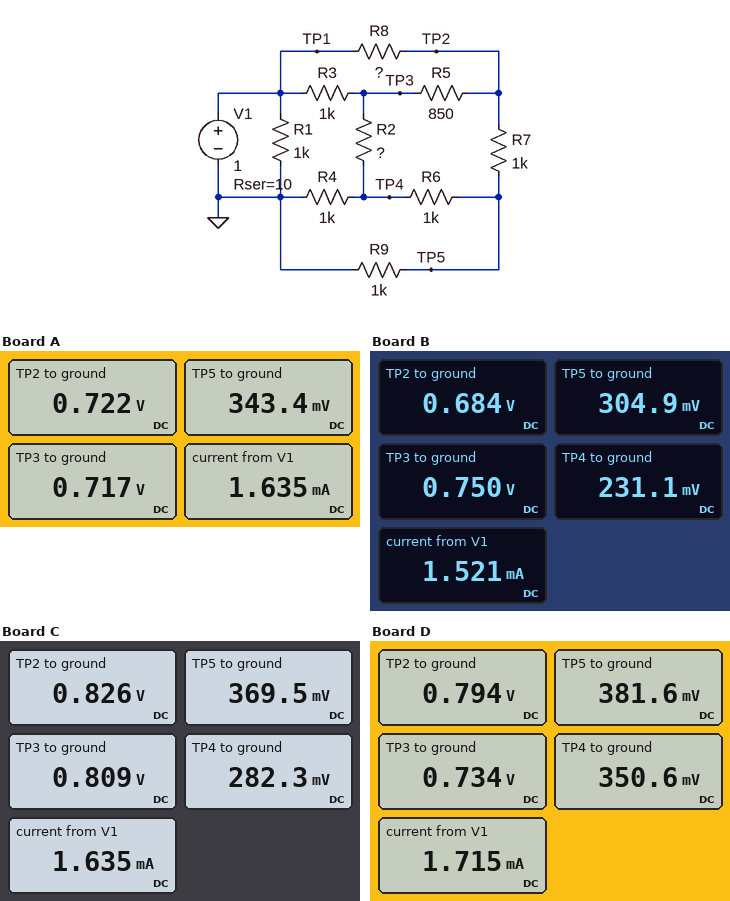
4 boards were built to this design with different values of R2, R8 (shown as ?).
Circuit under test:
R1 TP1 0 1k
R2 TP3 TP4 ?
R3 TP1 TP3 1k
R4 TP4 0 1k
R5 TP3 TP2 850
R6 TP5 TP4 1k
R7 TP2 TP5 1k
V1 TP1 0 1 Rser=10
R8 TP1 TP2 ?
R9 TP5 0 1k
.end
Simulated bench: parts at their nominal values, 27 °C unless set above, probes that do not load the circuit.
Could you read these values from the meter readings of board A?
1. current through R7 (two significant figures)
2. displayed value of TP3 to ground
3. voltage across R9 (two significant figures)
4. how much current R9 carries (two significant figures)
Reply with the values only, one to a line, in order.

380 µA
0.717 V
340 mV
340 µA
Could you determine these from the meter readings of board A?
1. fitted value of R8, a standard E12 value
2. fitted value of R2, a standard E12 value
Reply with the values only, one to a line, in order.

680 Ω
1.5 kΩ
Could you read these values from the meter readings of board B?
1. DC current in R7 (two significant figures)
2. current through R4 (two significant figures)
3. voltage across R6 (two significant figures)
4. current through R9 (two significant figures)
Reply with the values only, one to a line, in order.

380 µA
230 µA
74 mV
300 µA
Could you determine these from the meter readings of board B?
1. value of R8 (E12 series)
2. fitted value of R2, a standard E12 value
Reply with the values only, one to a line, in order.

1 kΩ
3.3 kΩ
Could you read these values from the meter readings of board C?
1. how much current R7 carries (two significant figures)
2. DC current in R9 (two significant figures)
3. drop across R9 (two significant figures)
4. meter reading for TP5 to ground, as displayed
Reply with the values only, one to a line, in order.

460 µA
370 µA
370 mV
369.5 mV
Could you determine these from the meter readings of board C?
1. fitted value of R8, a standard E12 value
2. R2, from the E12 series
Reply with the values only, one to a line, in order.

330 Ω
2.7 kΩ
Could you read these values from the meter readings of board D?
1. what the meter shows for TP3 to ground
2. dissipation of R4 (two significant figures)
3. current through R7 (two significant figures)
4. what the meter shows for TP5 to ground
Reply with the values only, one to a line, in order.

0.734 V
120 µW
410 µA
381.6 mV
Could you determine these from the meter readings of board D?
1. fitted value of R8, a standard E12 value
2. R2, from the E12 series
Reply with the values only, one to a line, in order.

390 Ω
1.2 kΩ
